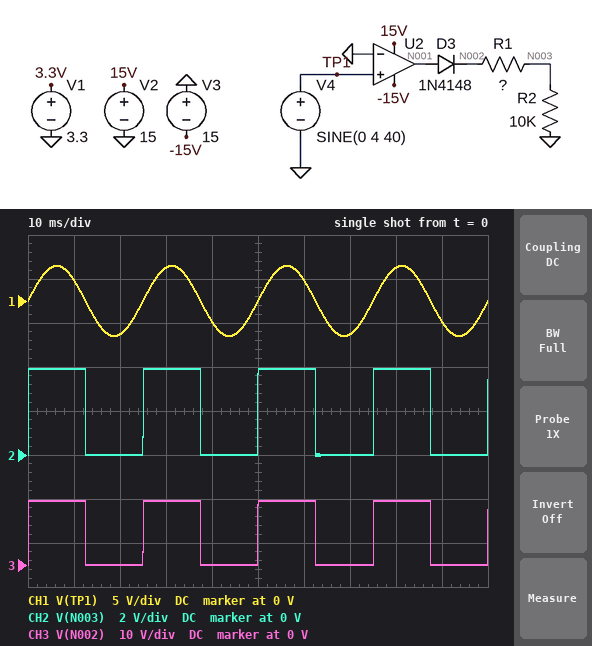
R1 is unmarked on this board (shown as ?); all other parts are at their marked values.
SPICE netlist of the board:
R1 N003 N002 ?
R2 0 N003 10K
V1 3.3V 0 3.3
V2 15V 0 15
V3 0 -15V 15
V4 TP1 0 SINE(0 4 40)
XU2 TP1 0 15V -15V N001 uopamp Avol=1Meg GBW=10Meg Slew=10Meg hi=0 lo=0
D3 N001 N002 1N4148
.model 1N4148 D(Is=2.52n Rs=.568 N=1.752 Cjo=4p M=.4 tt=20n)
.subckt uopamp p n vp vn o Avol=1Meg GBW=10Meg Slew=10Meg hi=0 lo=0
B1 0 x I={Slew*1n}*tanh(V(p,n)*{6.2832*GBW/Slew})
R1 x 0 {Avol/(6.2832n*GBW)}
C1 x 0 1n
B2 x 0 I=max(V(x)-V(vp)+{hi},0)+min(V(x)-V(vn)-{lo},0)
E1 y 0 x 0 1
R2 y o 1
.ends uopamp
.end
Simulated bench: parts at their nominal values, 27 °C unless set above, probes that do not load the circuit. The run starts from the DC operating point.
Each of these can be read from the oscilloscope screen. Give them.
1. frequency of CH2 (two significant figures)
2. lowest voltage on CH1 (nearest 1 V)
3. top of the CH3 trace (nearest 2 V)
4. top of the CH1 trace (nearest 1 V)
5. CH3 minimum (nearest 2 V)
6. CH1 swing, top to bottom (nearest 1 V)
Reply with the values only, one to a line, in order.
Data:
40 Hz
-4 V
14 V
4 V
0 V
8 V
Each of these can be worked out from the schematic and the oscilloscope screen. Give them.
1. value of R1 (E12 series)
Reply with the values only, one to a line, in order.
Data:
27 kΩ
